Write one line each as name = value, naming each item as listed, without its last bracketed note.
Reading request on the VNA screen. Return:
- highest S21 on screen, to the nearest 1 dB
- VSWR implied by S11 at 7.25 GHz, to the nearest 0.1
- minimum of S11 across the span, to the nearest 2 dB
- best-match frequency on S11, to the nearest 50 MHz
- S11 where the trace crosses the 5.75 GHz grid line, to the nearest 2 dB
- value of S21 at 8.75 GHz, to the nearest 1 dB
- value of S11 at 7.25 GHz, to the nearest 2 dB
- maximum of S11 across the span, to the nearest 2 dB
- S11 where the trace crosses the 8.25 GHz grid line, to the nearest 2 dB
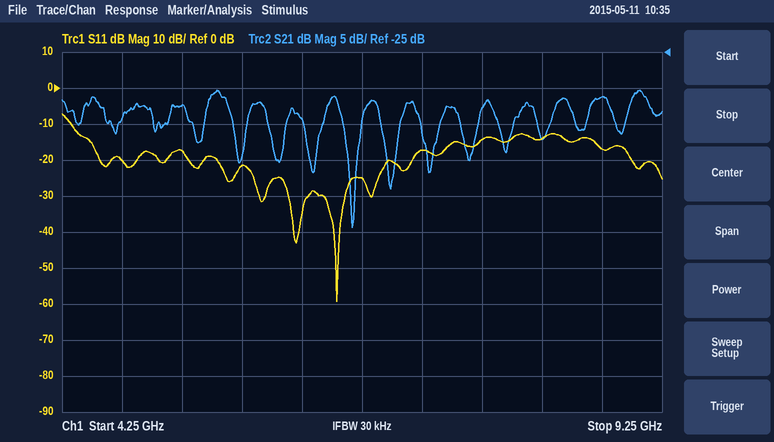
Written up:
highest S21 on screen, to the nearest 1 dB = -30 dB
VSWR implied by S11 at 7.25 GHz, to the nearest 0.1 = 1.3
minimum of S11 across the span, to the nearest 2 dB = -60 dB
best-match frequency on S11, to the nearest 50 MHz = 6.55 GHz
S11 where the trace crosses the 5.75 GHz grid line, to the nearest 2 dB = -22 dB
value of S21 at 8.75 GHz, to the nearest 1 dB = -31 dB
value of S11 at 7.25 GHz, to the nearest 2 dB = -18 dB
maximum of S11 across the span, to the nearest 2 dB = -8 dB
S11 where the trace crosses the 8.25 GHz grid line, to the nearest 2 dB = -14 dB
